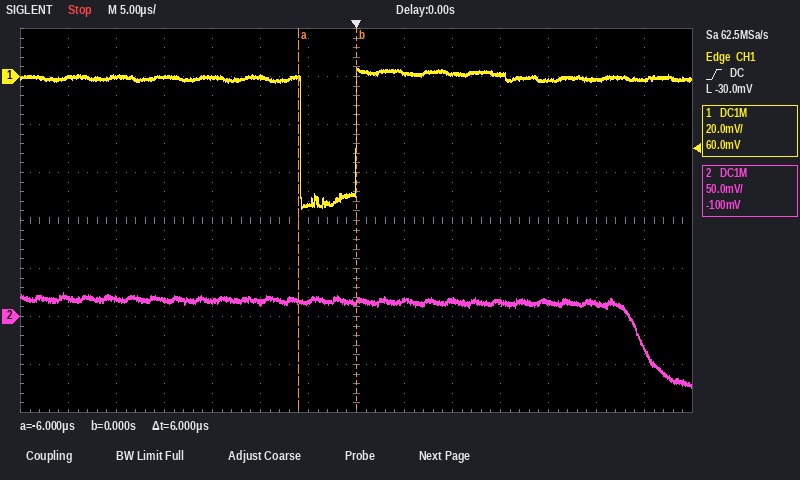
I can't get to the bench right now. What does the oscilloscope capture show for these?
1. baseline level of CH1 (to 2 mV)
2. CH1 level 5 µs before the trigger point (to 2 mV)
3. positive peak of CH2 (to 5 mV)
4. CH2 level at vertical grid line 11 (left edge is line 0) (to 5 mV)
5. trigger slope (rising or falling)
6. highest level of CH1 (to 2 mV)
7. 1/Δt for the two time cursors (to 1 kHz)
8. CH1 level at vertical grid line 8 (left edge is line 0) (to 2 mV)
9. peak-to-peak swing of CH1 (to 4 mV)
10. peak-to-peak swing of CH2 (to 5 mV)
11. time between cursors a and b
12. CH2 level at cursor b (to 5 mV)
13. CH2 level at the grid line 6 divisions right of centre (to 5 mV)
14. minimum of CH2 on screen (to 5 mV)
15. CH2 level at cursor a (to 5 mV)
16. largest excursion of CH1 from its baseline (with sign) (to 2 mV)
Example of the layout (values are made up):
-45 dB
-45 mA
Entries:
0 mV
-54 mV
25 mV
15 mV
rising
4 mV
167 kHz
2 mV
60 mV
100 mV
6 µs
15 mV
-35 mV
-75 mV
15 mV
-54 mV
